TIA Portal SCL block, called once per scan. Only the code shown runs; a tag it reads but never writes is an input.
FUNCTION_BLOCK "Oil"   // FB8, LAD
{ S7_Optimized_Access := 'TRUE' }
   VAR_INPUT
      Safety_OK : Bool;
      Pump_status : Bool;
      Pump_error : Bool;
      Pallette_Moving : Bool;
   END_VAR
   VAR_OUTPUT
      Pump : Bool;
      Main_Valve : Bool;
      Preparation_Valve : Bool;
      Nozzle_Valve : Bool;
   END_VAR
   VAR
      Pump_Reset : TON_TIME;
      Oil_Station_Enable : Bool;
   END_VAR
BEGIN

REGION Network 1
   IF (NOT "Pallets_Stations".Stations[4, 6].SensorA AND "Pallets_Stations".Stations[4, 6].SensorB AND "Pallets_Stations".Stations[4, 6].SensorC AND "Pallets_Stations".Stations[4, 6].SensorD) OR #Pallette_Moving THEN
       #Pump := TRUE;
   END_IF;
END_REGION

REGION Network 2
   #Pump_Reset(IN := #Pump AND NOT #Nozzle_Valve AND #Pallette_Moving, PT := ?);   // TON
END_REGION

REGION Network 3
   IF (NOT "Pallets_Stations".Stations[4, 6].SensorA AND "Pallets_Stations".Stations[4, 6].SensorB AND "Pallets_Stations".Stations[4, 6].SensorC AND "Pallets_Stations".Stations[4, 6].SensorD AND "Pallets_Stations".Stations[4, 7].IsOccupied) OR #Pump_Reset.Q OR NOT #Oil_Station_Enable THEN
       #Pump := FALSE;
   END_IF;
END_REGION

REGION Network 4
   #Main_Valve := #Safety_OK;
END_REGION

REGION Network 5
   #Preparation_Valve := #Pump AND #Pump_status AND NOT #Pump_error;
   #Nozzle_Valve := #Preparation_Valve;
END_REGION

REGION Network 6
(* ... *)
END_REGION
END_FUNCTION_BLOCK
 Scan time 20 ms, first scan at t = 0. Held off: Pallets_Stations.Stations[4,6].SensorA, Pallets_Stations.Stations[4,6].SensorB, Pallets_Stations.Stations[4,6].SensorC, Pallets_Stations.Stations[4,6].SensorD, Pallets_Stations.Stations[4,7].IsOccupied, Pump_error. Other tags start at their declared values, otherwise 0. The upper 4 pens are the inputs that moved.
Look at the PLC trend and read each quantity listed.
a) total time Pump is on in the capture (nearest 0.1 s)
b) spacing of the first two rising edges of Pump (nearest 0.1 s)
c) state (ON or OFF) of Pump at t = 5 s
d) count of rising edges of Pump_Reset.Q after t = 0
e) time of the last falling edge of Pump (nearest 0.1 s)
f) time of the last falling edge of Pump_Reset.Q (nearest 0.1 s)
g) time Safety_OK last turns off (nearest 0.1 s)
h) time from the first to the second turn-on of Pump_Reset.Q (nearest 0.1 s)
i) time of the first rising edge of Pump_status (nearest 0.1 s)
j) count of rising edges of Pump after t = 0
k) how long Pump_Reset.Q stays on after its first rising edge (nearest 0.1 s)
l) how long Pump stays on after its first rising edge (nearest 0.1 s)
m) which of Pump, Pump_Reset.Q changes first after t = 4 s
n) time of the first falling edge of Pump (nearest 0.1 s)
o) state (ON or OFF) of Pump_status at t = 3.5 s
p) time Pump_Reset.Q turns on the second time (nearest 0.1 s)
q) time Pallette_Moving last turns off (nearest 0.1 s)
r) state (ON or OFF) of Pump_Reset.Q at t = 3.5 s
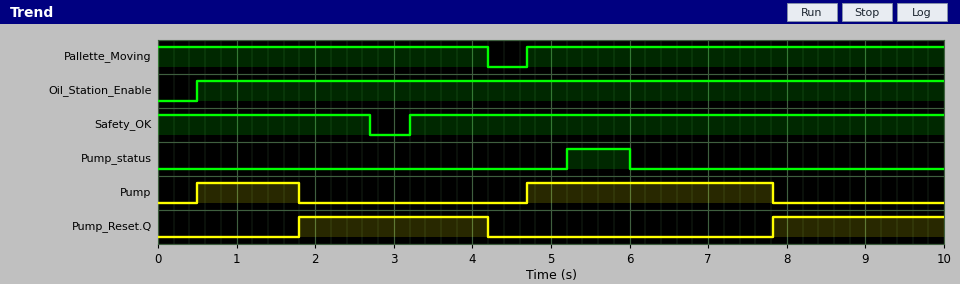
4.4 s
4.2 s
ON
2
7.8 s
4.2 s
2.7 s
6.0 s
5.2 s
2
2.4 s
1.3 s
Pump_Reset.Q
1.8 s
OFF
7.8 s
4.2 s
ON
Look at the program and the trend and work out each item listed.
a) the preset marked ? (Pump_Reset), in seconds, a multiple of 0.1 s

1.8 s
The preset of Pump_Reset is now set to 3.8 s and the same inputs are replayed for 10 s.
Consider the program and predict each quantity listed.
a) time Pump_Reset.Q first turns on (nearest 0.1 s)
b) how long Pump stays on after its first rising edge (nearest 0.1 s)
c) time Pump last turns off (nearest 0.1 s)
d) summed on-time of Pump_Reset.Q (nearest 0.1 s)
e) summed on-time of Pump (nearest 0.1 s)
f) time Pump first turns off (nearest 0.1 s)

3.8 s
3.3 s
9.8 s
0.6 s
8.4 s
3.8 s
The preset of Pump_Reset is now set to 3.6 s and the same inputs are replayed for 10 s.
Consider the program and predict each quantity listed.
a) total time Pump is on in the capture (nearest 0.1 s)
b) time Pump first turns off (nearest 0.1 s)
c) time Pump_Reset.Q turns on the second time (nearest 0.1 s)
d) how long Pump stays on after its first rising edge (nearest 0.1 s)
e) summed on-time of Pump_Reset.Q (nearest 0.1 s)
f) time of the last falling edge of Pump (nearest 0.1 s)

8.0 s
3.6 s
9.6 s
3.1 s
1.0 s
9.6 s
